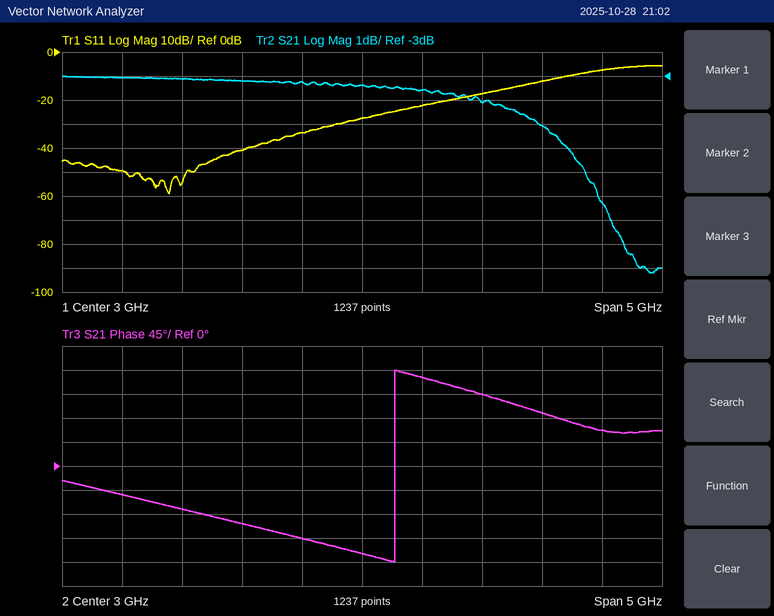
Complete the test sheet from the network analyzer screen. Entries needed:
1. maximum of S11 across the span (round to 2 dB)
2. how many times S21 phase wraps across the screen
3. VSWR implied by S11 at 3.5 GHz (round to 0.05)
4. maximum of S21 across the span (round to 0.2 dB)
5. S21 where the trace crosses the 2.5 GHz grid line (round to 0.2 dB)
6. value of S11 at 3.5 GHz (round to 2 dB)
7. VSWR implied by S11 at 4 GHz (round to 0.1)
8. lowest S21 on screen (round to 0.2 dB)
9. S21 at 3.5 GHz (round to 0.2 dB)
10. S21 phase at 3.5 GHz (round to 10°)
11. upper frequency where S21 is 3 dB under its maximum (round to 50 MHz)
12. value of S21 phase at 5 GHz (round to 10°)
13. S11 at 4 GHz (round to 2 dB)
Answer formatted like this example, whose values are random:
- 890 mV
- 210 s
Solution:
- -6 dB
- 1
- 1.15
- -3.0 dB
- -3.2 dB
- -22 dB
- 1.3
- -11.2 dB
- -3.6 dB
- 170°
- 4.70 GHz
- 70°
- -18 dB
